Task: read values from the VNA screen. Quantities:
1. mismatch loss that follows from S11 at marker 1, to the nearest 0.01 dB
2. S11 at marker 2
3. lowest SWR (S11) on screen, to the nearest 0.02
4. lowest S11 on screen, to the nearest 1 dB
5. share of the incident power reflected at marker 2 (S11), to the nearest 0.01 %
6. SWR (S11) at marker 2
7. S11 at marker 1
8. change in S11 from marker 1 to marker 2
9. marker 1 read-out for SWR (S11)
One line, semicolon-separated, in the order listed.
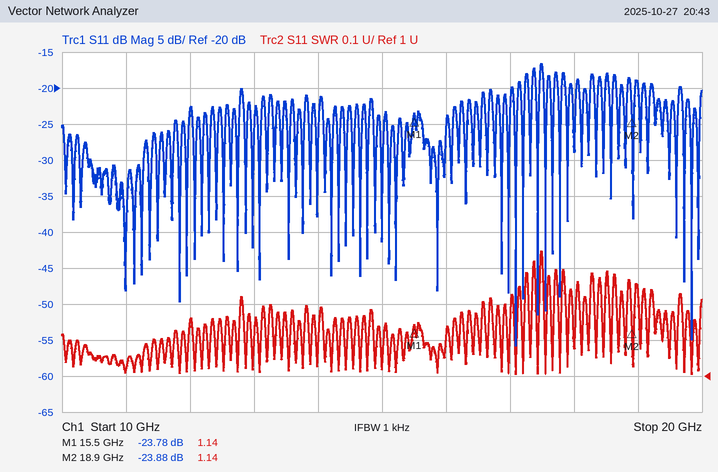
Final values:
0.02 dB; -23.88 dB; 1.00; -56 dB; 0.41 %; 1.14; -23.78 dB; -0.10 dB; 1.14
